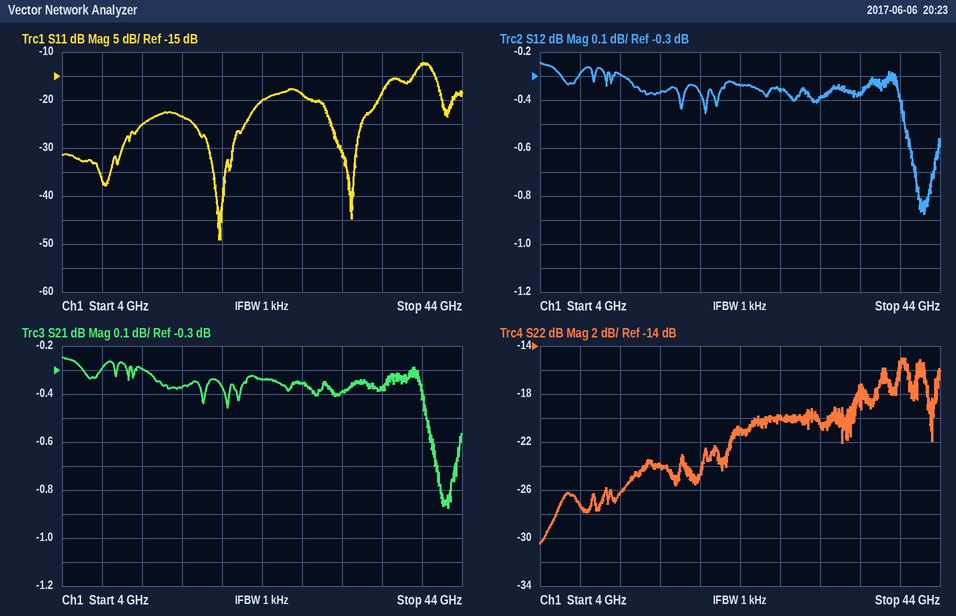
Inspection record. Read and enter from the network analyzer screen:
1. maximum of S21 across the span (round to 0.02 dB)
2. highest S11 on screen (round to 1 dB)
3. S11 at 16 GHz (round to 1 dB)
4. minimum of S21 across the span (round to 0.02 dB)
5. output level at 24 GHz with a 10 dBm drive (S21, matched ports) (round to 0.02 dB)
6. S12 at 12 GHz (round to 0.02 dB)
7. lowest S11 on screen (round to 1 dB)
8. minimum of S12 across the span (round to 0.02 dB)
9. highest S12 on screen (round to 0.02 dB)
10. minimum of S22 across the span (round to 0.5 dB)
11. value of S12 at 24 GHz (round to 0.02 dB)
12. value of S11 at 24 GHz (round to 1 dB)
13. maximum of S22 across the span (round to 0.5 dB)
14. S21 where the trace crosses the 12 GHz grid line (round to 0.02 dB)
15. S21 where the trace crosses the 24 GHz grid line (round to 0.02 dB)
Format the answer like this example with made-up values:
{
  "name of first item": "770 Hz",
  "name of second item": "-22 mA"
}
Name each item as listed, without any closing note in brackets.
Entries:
{
  "maximum of S21 across the span": "-0.24 dB",
  "highest S11 on screen": "-12 dB",
  "S11 at 16 GHz": "-23 dB",
  "minimum of S21 across the span": "-0.88 dB",
  "output level at 24 GHz with a 10 dBm drive (S21, matched ports)": "9.66 dBm",
  "S12 at 12 GHz": "-0.30 dB",
  "lowest S11 on screen": "-49 dB",
  "minimum of S12 across the span": "-0.88 dB",
  "highest S12 on screen": "-0.24 dB",
  "minimum of S22 across the span": "-30.5 dB",
  "value of S12 at 24 GHz": "-0.34 dB",
  "value of S11 at 24 GHz": "-20 dB",
  "maximum of S22 across the span": "-15.0 dB",
  "S21 where the trace crosses the 12 GHz grid line": "-0.30 dB",
  "S21 where the trace crosses the 24 GHz grid line": "-0.34 dB"
}
